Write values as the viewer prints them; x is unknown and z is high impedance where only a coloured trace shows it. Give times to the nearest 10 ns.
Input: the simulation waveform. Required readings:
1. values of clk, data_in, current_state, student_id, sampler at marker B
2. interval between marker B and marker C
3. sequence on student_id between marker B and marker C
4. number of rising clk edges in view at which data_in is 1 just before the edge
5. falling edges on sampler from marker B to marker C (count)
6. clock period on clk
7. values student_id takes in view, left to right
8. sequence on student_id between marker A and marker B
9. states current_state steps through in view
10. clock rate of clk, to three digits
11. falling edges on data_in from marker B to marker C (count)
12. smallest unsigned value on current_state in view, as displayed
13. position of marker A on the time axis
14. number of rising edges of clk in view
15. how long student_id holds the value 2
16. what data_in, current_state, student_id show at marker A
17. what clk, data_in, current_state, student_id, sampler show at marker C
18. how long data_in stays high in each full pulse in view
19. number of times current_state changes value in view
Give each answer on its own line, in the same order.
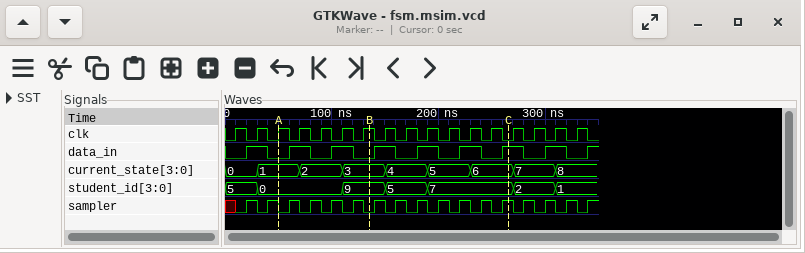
clk=1, data_in=0, current_state=3, student_id=9, sampler=0
130 ns
9, 5, 7
8
6
20 ns
5, 0, 9, 5, 7, 2, 1
0, 9
0, 1, 2, 3, 4, 5, 6, 7, 8
50.0 MHz
3
0
50 ns
17
40 ns
data_in=0, current_state=1, student_id=0
clk=0, data_in=1, current_state=6, student_id=7, sampler=1
20 ns, 20 ns, 20 ns, 20 ns, 20 ns, 20 ns, 20 ns, 20 ns
8
